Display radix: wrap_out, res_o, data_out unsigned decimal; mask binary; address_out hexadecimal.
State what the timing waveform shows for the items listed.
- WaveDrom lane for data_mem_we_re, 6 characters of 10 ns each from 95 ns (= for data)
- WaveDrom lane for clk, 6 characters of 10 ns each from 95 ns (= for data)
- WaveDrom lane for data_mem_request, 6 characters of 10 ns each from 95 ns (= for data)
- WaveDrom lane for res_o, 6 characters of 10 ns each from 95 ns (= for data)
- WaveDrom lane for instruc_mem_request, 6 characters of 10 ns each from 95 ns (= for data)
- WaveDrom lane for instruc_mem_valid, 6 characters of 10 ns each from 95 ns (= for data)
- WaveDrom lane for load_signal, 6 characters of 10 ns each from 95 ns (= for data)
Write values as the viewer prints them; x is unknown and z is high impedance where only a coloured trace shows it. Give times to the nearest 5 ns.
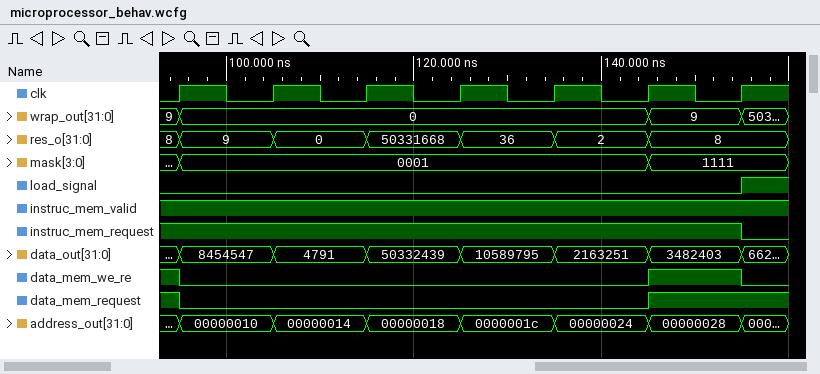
{name: 'data_mem_we_re', wave: '0....1'}
{name: 'clk', wave: 'p.....'}
{name: 'data_mem_request', wave: '0....1'}
{name: 'res_o', wave: '======', data: '9 0 50331668 36 2 8'}
{name: 'instruc_mem_request', wave: '1.....'}
{name: 'instruc_mem_valid', wave: '1.....'}
{name: 'load_signal', wave: '0.....'}
